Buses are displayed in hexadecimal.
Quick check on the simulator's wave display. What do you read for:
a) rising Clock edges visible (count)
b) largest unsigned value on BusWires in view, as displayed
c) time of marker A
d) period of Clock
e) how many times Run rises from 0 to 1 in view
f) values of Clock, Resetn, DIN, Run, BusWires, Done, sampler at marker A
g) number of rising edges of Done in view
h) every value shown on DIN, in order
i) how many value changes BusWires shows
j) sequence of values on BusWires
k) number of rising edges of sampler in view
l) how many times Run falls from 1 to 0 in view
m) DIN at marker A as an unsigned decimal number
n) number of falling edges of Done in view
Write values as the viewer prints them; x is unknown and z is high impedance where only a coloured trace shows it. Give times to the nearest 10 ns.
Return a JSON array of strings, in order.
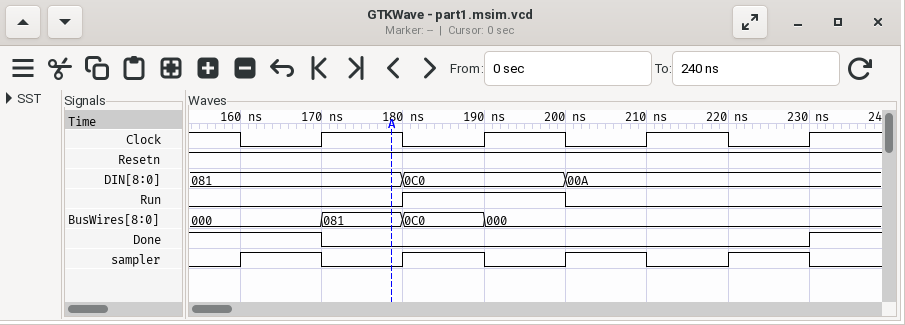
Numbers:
["4", "0C0", "180 ns", "20 ns", "1", "Clock=1, Resetn=1, DIN=081, Run=0, BusWires=081, Done=0, sampler=0", "1", "081, 0C0, 00A", "3", "000, 081, 0C0, 000", "4", "1", "129", "1"]
